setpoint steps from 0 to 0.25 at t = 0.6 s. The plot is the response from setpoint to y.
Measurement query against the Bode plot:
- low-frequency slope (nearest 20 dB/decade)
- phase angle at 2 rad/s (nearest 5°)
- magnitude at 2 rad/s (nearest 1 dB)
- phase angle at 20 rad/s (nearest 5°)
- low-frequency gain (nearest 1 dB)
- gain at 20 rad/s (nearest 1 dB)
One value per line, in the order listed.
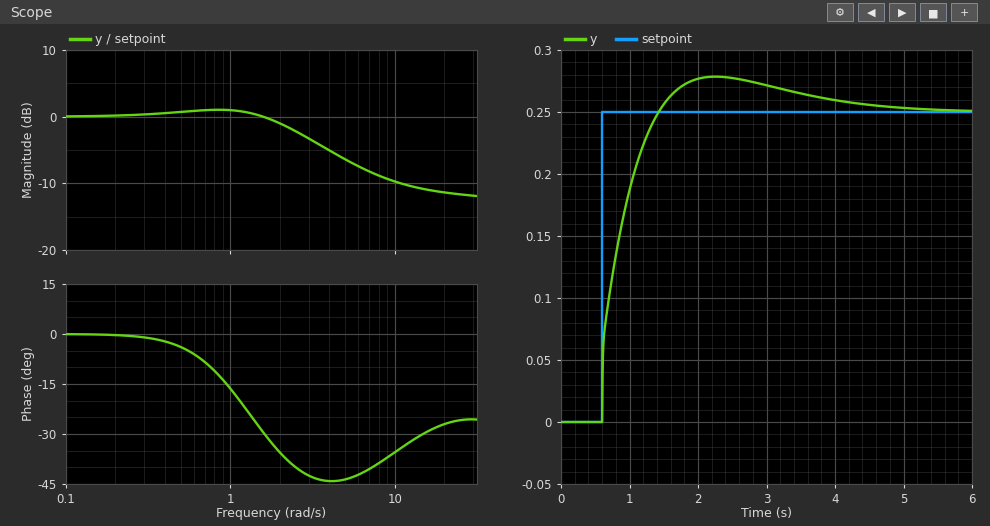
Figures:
0 dB/decade
-35°
-1 dB
-25°
0 dB
-11 dB
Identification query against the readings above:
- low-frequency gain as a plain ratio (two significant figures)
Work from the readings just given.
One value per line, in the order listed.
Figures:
1.0
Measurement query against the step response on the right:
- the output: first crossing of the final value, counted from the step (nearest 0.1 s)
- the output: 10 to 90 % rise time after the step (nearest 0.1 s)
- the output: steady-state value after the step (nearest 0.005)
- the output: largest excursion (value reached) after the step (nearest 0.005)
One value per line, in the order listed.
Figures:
0.8 s
0.6 s
0.250
0.280
